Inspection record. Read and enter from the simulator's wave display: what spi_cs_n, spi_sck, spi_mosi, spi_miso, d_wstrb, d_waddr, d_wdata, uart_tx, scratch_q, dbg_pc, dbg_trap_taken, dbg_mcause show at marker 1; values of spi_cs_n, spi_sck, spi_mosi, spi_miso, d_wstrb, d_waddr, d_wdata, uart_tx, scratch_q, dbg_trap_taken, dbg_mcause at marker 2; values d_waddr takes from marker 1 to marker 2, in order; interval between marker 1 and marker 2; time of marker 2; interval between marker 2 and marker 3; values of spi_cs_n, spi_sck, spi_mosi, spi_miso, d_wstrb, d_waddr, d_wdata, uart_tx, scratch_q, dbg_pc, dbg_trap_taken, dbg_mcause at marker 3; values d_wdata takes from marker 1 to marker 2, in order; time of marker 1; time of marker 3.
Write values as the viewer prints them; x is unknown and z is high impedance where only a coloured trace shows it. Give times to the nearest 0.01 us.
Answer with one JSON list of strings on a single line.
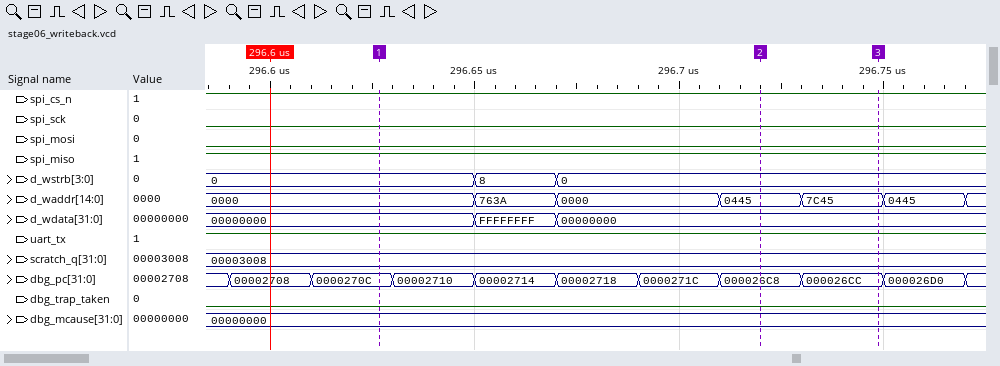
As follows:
["spi_cs_n=1, spi_sck=0, spi_mosi=0, spi_miso=1, d_wstrb=0, d_waddr=0000, d_wdata=00000000, uart_tx=1, scratch_q=00003008, dbg_pc=0000270C, dbg_trap_taken=0, dbg_mcause=00000000", "spi_cs_n=1, spi_sck=0, spi_mosi=0, spi_miso=1, d_wstrb=0, d_waddr=0445, d_wdata=00000000, uart_tx=1, scratch_q=00003008, dbg_trap_taken=0, dbg_mcause=00000000", "0000, 763A, 0000, 0445", "0.09 us", "296.72 us", "0.03 us", "spi_cs_n=1, spi_sck=0, spi_mosi=0, spi_miso=1, d_wstrb=0, d_waddr=7C45, d_wdata=00000000, uart_tx=1, scratch_q=00003008, dbg_pc=000026CC, dbg_trap_taken=0, dbg_mcause=00000000", "00000000, FFFFFFFF, 00000000", "296.63 us", "296.75 us"]
